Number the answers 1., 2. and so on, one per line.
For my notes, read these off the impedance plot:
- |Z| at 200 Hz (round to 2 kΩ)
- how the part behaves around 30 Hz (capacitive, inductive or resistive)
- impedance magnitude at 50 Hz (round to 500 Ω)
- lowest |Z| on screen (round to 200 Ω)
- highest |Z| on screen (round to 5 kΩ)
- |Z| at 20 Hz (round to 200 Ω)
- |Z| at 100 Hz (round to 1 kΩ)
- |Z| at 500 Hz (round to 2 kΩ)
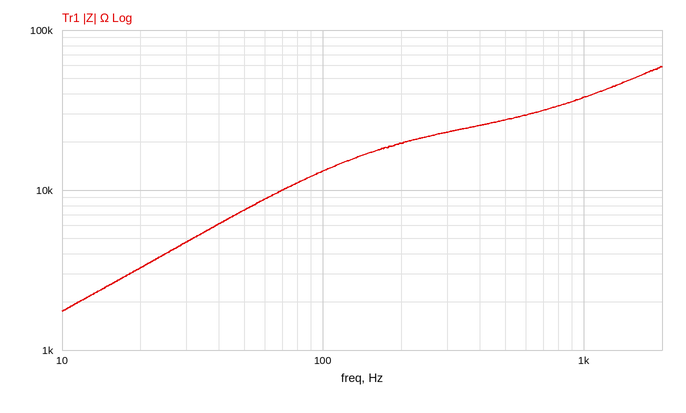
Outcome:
1. 20 kΩ
2. inductive
3. 7.5 kΩ
4. 1.8 kΩ
5. 60 kΩ
6. 3.2 kΩ
7. 13 kΩ
8. 28 kΩ
